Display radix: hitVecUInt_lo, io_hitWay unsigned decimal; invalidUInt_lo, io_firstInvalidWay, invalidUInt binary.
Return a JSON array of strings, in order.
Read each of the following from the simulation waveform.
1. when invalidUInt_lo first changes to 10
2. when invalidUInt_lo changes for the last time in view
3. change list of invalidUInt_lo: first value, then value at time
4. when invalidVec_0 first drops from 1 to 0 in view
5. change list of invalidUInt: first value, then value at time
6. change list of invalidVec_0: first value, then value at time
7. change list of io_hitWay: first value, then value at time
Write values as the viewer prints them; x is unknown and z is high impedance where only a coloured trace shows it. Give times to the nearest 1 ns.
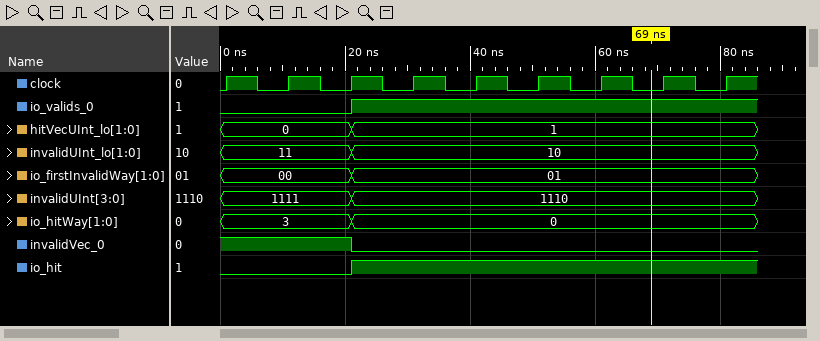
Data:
["21 ns", "21 ns", "11, 10 at 21 ns", "21 ns", "1111, 1110 at 21 ns", "1, 0 at 21 ns", "3, 0 at 21 ns"]
